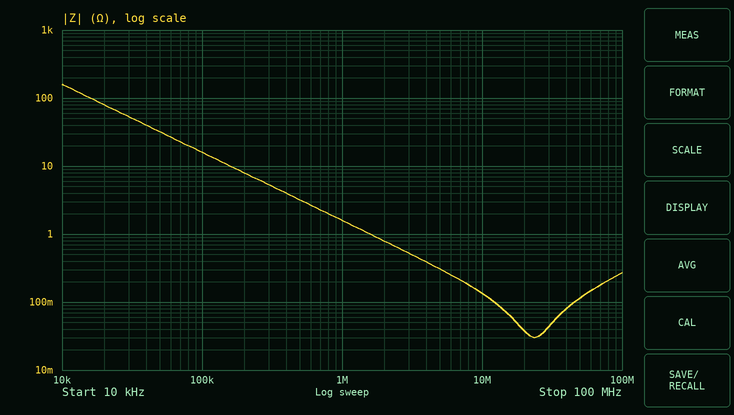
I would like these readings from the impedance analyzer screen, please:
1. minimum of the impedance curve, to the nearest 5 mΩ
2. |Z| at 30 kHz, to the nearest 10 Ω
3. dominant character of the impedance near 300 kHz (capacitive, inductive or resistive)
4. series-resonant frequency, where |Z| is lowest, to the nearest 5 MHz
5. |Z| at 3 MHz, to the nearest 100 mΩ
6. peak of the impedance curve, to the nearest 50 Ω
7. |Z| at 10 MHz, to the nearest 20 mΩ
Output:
30 mΩ
50 Ω
capacitive
25 MHz
500 mΩ
150 Ω
140 mΩ
